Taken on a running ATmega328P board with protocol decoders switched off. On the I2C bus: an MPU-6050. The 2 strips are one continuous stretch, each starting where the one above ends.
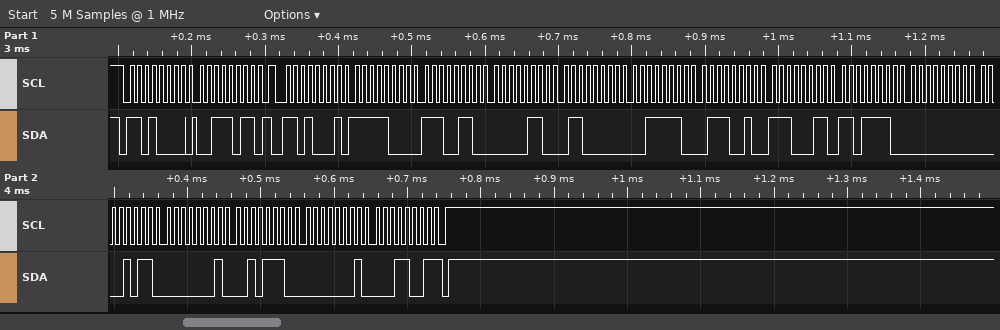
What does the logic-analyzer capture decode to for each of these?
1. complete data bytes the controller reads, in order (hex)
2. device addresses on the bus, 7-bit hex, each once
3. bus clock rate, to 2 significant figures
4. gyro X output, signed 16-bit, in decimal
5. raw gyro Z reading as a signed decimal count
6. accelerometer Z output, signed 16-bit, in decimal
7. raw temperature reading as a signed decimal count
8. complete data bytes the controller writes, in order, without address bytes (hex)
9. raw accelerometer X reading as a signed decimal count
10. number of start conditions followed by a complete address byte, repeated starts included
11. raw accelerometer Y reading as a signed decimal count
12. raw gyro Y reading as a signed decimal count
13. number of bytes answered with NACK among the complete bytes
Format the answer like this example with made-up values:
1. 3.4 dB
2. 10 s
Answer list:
1. F8 E6 06 60 3E 72 E3 DE 00 0B 01 2E 01 19
2. 0x68
3. 100 kHz
4. 11
5. 281
6. 15986
7. -7202
8. 3B
9. -1818
10. 2
11. 1632
12. 302
13. 1
